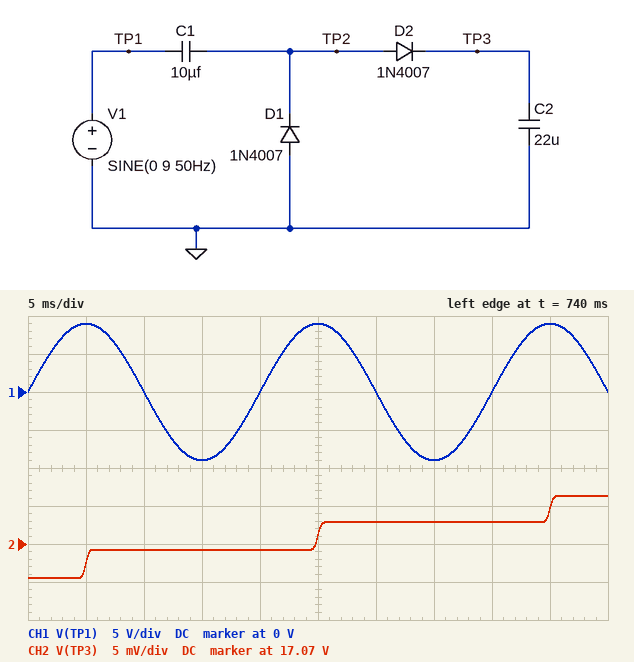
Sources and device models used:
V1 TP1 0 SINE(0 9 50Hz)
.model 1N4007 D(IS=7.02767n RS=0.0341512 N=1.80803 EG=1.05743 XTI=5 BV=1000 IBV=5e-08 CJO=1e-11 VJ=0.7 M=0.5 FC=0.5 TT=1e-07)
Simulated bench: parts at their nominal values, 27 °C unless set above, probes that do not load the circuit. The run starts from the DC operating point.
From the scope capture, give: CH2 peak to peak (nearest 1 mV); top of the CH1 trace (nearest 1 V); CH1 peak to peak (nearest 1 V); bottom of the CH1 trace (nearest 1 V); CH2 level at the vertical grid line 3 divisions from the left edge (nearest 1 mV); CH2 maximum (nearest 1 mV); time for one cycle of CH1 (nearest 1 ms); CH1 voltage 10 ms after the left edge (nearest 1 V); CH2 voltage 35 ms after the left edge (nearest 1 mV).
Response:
11 mV
9 V
18 V
-9 V
17.064 V
17.071 V
20 ms
0 V
17.068 V
